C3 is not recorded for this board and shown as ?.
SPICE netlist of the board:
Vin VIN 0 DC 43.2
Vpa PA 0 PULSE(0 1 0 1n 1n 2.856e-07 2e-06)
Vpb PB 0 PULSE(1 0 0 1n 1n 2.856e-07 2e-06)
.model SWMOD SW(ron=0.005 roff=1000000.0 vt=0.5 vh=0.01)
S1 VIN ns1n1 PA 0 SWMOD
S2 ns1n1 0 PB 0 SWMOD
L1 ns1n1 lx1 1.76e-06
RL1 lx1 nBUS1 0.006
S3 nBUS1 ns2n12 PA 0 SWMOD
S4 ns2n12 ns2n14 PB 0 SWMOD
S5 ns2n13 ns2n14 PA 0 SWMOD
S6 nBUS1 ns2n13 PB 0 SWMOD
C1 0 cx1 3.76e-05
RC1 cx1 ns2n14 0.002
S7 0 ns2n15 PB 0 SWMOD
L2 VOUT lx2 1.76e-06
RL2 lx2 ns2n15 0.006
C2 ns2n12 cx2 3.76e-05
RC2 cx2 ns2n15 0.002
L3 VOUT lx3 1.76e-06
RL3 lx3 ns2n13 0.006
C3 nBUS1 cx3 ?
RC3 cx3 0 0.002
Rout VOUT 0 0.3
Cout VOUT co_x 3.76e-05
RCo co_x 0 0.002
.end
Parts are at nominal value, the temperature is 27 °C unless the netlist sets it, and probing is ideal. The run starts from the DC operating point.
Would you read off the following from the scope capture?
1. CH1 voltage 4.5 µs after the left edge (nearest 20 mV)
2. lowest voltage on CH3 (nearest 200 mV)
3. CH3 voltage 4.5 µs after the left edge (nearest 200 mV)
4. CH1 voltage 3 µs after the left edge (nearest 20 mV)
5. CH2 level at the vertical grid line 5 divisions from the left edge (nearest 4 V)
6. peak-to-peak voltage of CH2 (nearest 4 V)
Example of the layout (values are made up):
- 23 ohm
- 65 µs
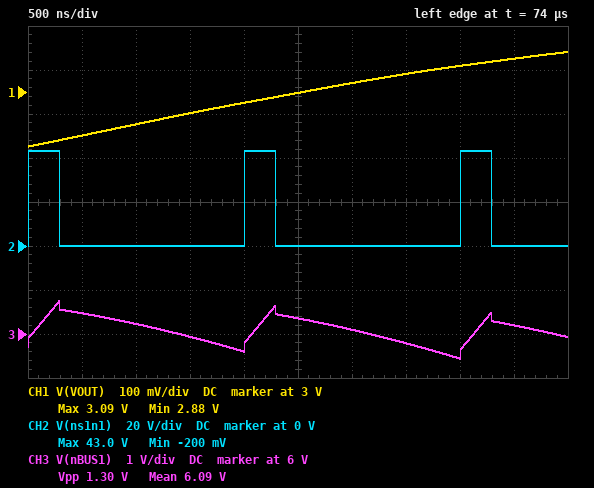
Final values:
- 3.08 V
- 5.4 V
- 6.2 V
- 3.02 V
- 0 V
- 44 V
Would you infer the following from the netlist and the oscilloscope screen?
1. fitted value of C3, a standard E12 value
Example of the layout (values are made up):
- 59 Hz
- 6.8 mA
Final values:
- 27 µF
